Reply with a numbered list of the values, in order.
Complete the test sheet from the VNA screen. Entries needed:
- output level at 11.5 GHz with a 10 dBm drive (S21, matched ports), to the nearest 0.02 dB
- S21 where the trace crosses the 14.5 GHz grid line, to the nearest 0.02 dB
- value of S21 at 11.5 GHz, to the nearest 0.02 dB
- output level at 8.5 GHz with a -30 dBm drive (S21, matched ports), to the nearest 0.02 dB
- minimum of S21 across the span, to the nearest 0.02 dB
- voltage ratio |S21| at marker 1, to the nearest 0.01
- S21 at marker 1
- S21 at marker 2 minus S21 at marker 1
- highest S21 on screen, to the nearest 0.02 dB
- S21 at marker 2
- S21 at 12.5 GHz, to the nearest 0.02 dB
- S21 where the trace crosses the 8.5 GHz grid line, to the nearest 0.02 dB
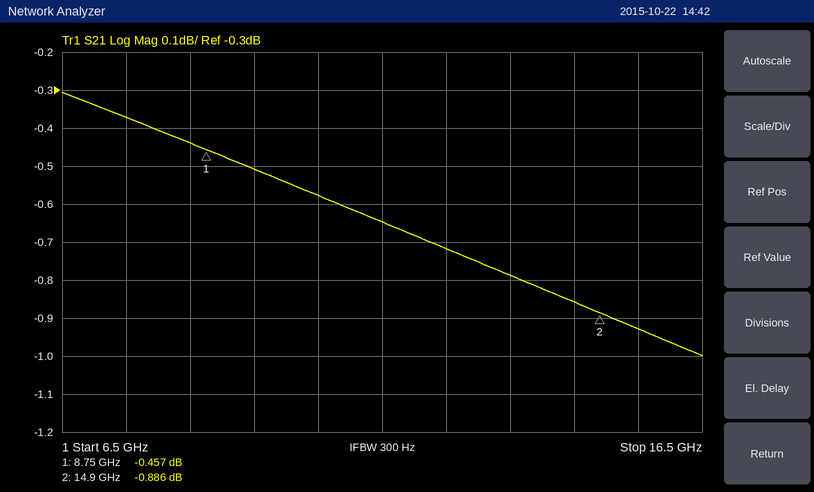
1. 9.36 dBm
2. -0.86 dB
3. -0.64 dB
4. -30.44 dBm
5. -1.00 dB
6. 0.95
7. -0.457 dB
8. -0.429 dB
9. -0.30 dB
10. -0.886 dB
11. -0.72 dB
12. -0.44 dB
